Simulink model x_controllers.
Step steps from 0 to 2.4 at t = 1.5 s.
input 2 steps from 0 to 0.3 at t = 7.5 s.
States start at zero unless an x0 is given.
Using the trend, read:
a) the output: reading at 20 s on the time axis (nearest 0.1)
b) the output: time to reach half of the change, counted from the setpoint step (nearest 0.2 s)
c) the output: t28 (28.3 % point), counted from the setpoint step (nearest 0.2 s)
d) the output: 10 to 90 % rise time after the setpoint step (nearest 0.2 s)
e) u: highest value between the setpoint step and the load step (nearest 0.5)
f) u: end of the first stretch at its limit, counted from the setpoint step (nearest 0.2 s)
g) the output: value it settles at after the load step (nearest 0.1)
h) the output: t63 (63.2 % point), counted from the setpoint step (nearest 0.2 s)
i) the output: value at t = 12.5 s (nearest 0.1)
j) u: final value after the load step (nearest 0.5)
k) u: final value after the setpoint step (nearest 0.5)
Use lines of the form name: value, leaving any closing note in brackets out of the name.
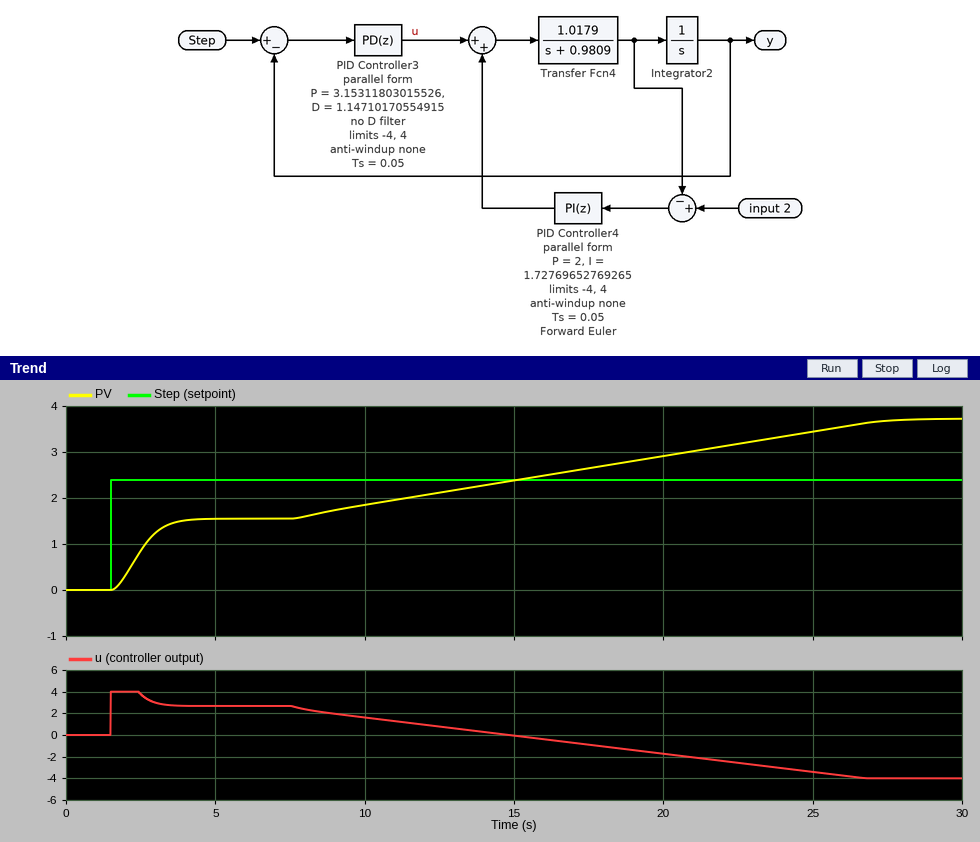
the output: reading at 20 s on the time axis: 2.9
the output: time to reach half of the change, counted from the setpoint step: 1.0 s
the output: t28 (28.3 % point), counted from the setpoint step: 0.6 s
the output: 10 to 90 % rise time after the setpoint step: 1.6 s
u: highest value between the setpoint step and the load step: 4.0
u: end of the first stretch at its limit, counted from the setpoint step: 1.0 s
the output: value it settles at after the load step: 3.7
the output: t63 (63.2 % point), counted from the setpoint step: 1.2 s
the output: value at t = 12.5 s: 2.1
u: final value after the load step: -4.0
u: final value after the setpoint step: 2.5
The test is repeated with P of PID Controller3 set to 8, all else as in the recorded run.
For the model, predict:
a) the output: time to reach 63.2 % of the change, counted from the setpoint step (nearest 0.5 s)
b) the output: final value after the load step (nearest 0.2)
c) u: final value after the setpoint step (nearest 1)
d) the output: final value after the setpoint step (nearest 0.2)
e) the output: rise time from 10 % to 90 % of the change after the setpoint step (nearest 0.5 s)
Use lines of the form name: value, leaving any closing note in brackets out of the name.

the output: time to reach 63.2 % of the change, counted from the setpoint step: 1.5 s
the output: final value after the load step: 3.0
u: final value after the setpoint step: 3
the output: final value after the setpoint step: 2.0
the output: rise time from 10 % to 90 % of the change after the setpoint step: 2.0 s
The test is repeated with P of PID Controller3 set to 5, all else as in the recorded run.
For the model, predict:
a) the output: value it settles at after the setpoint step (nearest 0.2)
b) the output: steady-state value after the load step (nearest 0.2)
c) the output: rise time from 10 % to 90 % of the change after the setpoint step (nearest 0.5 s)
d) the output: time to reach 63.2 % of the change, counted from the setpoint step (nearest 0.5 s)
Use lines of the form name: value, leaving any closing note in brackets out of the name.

the output: value it settles at after the setpoint step: 1.8
the output: steady-state value after the load step: 3.2
the output: rise time from 10 % to 90 % of the change after the setpoint step: 1.5 s
the output: time to reach 63.2 % of the change, counted from the setpoint step: 1.5 s
